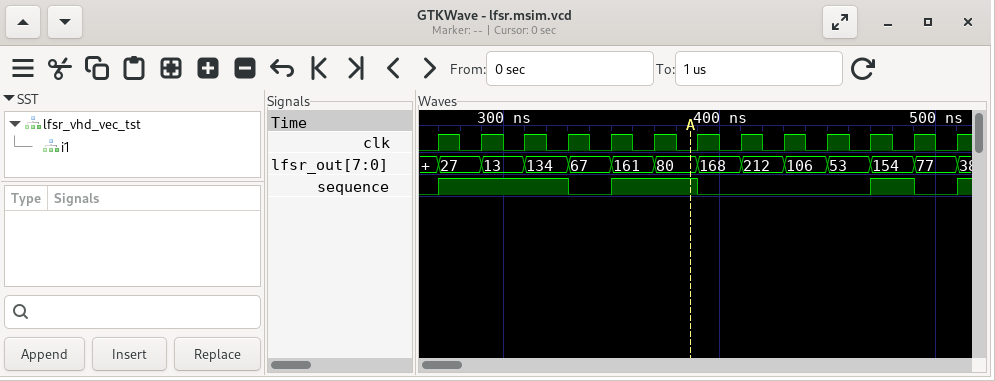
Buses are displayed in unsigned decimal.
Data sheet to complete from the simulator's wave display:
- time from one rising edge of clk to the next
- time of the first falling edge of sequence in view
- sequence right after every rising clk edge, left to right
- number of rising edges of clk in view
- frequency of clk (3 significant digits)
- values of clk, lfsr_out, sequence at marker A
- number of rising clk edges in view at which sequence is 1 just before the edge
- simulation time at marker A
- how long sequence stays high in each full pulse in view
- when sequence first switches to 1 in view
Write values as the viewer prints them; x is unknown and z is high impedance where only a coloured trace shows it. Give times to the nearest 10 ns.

20 ns
330 ns
1 1 1 0 1 1 0 0 0 0 1 0 1
13
50.0 MHz
clk=0, lfsr_out=80, sequence=1
6
390 ns
60 ns, 40 ns, 20 ns
270 ns
